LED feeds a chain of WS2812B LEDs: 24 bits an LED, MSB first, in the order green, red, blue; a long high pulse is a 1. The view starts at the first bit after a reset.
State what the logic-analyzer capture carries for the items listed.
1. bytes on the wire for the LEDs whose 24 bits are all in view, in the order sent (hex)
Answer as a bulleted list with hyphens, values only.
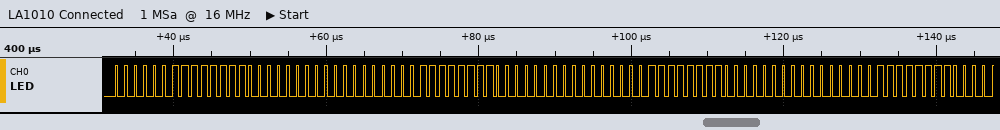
- 03 FC 00 00 FF 00 00 FF 00
